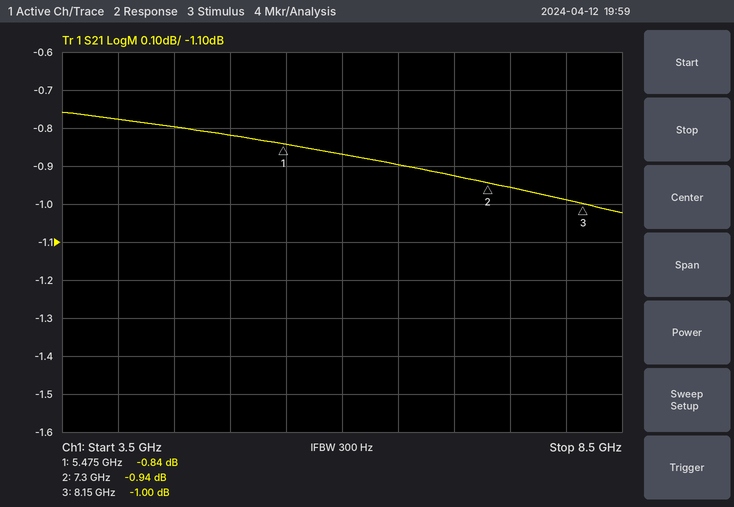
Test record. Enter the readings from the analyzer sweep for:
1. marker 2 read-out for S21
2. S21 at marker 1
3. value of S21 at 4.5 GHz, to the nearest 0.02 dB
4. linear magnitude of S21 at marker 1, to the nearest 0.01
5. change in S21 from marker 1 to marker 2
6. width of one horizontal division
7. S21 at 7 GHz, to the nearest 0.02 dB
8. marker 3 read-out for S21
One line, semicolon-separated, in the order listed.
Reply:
-0.94 dB; -0.84 dB; -0.80 dB; 0.91; -0.10 dB; 500 MHz; -0.92 dB; -1.00 dB
